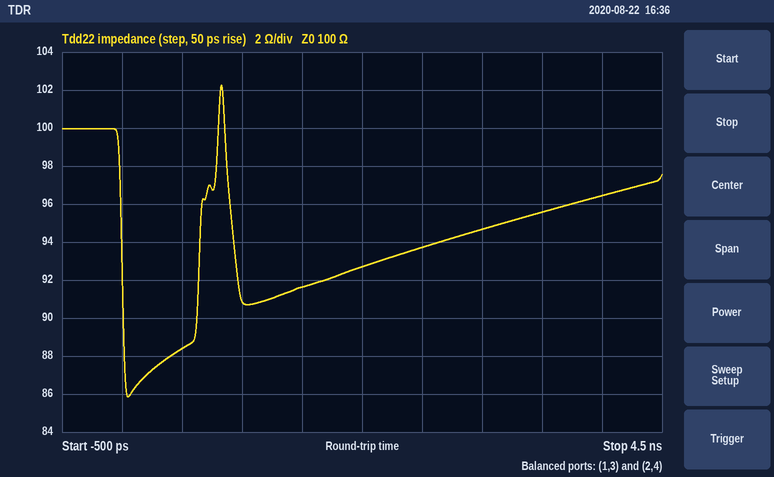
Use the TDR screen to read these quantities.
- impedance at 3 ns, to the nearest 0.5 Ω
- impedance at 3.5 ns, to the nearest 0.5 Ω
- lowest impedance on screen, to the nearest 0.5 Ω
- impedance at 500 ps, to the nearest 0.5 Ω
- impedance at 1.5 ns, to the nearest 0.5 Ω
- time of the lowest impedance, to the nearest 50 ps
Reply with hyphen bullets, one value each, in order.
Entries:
- 94.5 Ω
- 95.5 Ω
- 86.0 Ω
- 88.5 Ω
- 91.5 Ω
- 50 ps
